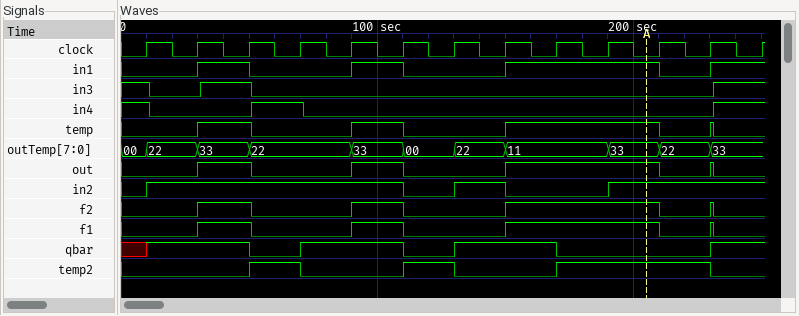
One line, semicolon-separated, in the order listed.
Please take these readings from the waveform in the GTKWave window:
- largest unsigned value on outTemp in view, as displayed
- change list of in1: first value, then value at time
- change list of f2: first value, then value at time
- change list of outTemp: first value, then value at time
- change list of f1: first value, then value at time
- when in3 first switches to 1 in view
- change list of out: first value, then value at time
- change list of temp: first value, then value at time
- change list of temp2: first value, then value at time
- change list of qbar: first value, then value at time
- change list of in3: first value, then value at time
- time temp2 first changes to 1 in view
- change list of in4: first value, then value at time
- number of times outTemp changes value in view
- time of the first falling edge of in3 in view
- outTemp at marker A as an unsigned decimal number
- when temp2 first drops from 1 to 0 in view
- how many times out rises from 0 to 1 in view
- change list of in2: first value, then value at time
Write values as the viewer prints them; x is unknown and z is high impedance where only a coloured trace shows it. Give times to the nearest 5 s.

33; 0, 1 at 30 s, 0 at 50 s, 1 at 90 s, 0 at 110 s, 1 at 150 s, 0 at 210 s, 1 at 230 s; 0, 1 at 30 s, 0 at 50 s, 1 at 90 s, 0 at 110 s, 1 at 150 s, 0 at 210 s, 1 at 230 s, 0 at 230 s; 00, 22 at 10 s, 33 at 30 s, 22 at 50 s, 33 at 90 s, 00 at 110 s, 22 at 130 s, 11 at 150 s, 33 at 190 s, 22 at 210 s, 33 at 230 s; 0, 1 at 30 s, 0 at 50 s, 1 at 90 s, 0 at 110 s, 1 at 150 s, 0 at 210 s, 1 at 230 s, 0 at 230 s; 30 s; 0, 1 at 30 s, 0 at 50 s, 1 at 90 s, 0 at 110 s, 1 at 150 s, 0 at 210 s, 1 at 230 s, 0 at 230 s; 0, 1 at 30 s, 0 at 50 s, 1 at 90 s, 0 at 110 s, 1 at 150 s, 0 at 210 s, 1 at 230 s, 0 at 230 s; 0, 1 at 50 s, 0 at 70 s, 1 at 110 s, 0 at 130 s, 1 at 170 s, 0 at 230 s; x, 1 at 10 s, 0 at 50 s, 1 at 70 s, 0 at 110 s, 1 at 130 s, 0 at 170 s, 1 at 230 s; 1, 0 at 10 s, 1 at 30 s, 0 at 50 s, 1 at 230 s; 50 s; 1, 0 at 10 s, 1 at 50 s, 0 at 70 s, 1 at 230 s; 10; 10 s; 51; 70 s; 4; 0, 1 at 10 s, 0 at 110 s, 1 at 130 s, 0 at 150 s, 1 at 190 s
